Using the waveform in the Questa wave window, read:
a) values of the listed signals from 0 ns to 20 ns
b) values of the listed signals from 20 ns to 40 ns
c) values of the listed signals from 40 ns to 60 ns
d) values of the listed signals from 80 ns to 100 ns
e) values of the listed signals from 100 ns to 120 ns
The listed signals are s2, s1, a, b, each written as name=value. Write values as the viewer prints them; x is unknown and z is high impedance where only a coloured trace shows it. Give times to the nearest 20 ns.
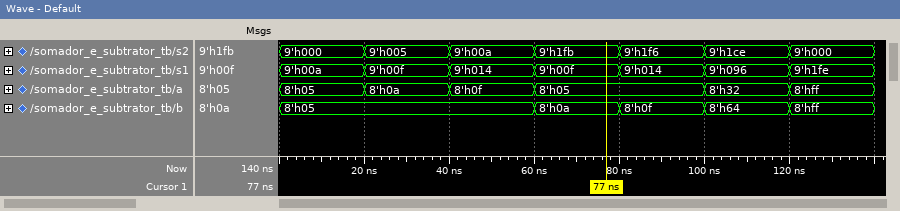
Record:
s2=9'h000, s1=9'h00a, a=8'h05, b=8'h05
s2=9'h005, s1=9'h00f, a=8'h0a, b=8'h05
s2=9'h00a, s1=9'h014, a=8'h0f, b=8'h05
s2=9'h1f6, s1=9'h014, a=8'h05, b=8'h0f
s2=9'h1ce, s1=9'h096, a=8'h32, b=8'h64
